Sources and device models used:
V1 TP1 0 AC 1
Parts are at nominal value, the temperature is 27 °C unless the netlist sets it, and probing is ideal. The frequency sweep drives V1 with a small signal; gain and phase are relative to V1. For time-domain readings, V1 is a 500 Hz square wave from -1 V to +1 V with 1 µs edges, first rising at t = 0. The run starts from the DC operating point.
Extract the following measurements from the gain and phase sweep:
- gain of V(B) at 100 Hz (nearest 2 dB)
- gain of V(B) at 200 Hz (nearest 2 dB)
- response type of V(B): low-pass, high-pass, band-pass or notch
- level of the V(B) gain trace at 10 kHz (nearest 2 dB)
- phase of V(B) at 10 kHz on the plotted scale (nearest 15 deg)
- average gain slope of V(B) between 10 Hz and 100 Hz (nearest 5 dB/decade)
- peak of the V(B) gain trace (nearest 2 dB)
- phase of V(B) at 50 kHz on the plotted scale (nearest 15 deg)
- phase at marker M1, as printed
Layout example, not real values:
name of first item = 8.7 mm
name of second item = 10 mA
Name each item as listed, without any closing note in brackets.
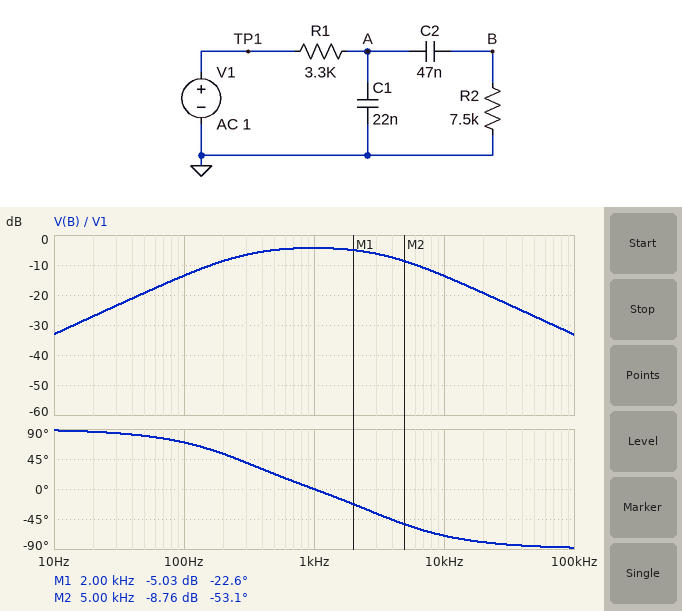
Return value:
gain of V(B) at 100 Hz = -14 dB
gain of V(B) at 200 Hz = -8 dB
response type of V(B): low-pass, high-pass, band-pass or notch = band-pass
level of the V(B) gain trace at 10 kHz = -14 dB
phase of V(B) at 10 kHz on the plotted scale = -75 deg
average gain slope of V(B) between 10 Hz and 100 Hz = 20 dB/decade
peak of the V(B) gain trace = -4 dB
phase of V(B) at 50 kHz on the plotted scale = -90 deg
phase at marker M1, as printed = -22.6 deg
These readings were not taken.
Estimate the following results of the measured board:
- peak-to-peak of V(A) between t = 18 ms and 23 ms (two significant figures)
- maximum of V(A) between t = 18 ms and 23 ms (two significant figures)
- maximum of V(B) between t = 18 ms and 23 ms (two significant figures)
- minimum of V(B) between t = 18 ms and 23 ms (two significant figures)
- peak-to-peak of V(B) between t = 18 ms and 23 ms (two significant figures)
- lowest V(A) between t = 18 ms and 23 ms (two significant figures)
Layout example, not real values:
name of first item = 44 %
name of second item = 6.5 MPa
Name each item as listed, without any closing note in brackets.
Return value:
peak-to-peak of V(A) between t = 18 ms and 23 ms = 1.8 V
maximum of V(A) between t = 18 ms and 23 ms = 900 mV
maximum of V(B) between t = 18 ms and 23 ms = 890 mV
minimum of V(B) between t = 18 ms and 23 ms = -890 mV
peak-to-peak of V(B) between t = 18 ms and 23 ms = 1.8 V
lowest V(A) between t = 18 ms and 23 ms = -900 mV
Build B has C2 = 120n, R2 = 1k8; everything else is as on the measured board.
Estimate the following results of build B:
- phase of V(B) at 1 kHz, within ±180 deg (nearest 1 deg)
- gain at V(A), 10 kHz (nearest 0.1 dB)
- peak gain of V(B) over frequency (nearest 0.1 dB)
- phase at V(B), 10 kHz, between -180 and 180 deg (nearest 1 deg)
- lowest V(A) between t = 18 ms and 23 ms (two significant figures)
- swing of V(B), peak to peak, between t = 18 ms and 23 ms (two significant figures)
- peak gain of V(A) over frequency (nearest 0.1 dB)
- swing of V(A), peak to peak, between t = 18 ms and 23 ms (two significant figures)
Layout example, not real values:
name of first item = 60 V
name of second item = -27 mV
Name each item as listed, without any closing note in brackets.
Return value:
phase of V(B) at 1 kHz, within ±180 deg = 5 deg
gain at V(A), 10 kHz = -14.8 dB
peak gain of V(B) over frequency = -10.0 dB
phase at V(B), 10 kHz, between -180 and 180 deg = -55 deg
lowest V(A) between t = 18 ms and 23 ms = -750 mV
swing of V(B), peak to peak, between t = 18 ms and 23 ms = 940 mV
peak gain of V(A) over frequency = 0 dB
swing of V(A), peak to peak, between t = 18 ms and 23 ms = 1.5 V
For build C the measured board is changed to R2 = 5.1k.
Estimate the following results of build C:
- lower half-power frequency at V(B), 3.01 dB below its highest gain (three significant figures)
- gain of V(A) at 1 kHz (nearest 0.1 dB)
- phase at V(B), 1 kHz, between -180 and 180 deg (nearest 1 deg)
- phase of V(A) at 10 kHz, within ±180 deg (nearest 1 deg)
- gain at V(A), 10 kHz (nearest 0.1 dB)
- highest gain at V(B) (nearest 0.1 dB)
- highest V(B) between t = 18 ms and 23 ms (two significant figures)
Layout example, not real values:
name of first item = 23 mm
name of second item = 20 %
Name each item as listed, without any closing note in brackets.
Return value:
lower half-power frequency at V(B), 3.01 dB below its highest gain = 317 Hz
gain of V(A) at 1 kHz = -4.3 dB
phase at V(B), 1 kHz, between -180 and 180 deg = 6 deg
phase of V(A) at 10 kHz, within ±180 deg = -70 deg
gain at V(A), 10 kHz = -13.8 dB
highest gain at V(B) = -5.8 dB
highest V(B) between t = 18 ms and 23 ms = 790 mV
